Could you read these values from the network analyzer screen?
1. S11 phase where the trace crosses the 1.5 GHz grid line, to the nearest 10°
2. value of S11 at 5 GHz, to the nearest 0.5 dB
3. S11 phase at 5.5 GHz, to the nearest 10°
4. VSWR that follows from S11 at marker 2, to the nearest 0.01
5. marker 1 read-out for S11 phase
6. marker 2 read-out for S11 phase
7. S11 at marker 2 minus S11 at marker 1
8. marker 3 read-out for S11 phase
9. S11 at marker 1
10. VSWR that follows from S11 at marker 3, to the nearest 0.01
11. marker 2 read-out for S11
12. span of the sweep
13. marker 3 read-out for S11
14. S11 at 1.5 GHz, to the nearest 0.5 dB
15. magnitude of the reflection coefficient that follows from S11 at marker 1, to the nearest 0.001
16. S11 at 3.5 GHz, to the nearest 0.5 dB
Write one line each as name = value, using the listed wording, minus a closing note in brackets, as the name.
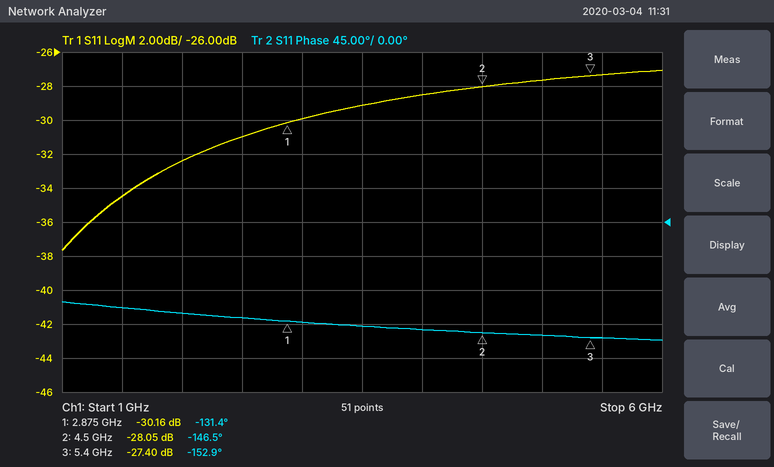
S11 phase where the trace crosses the 1.5 GHz grid line, to the nearest 10° = -110°
value of S11 at 5 GHz, to the nearest 0.5 dB = -27.5 dB
S11 phase at 5.5 GHz, to the nearest 10° = -150°
VSWR that follows from S11 at marker 2, to the nearest 0.01 = 1.08
marker 1 read-out for S11 phase = -131.4°
marker 2 read-out for S11 phase = -146.5°
S11 at marker 2 minus S11 at marker 1 = 2.11 dB
marker 3 read-out for S11 phase = -152.9°
S11 at marker 1 = -30.16 dB
VSWR that follows from S11 at marker 3, to the nearest 0.01 = 1.09
marker 2 read-out for S11 = -28.05 dB
span of the sweep = 5 GHz
marker 3 read-out for S11 = -27.40 dB
S11 at 1.5 GHz, to the nearest 0.5 dB = -34.5 dB
magnitude of the reflection coefficient that follows from S11 at marker 1, to the nearest 0.001 = 0.031
S11 at 3.5 GHz, to the nearest 0.5 dB = -29.0 dB
